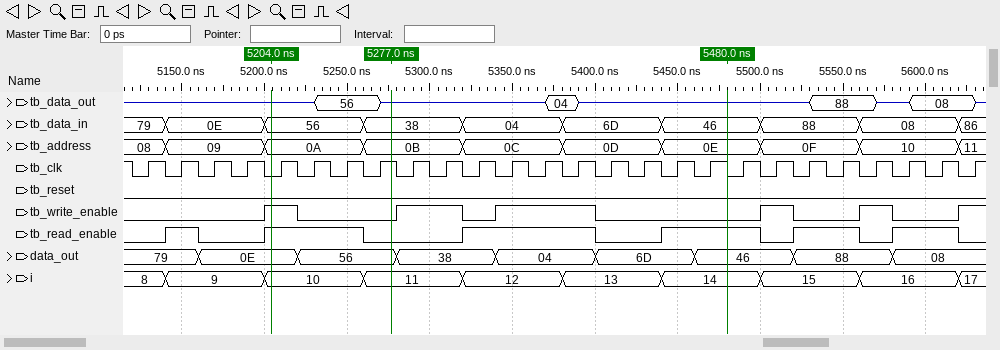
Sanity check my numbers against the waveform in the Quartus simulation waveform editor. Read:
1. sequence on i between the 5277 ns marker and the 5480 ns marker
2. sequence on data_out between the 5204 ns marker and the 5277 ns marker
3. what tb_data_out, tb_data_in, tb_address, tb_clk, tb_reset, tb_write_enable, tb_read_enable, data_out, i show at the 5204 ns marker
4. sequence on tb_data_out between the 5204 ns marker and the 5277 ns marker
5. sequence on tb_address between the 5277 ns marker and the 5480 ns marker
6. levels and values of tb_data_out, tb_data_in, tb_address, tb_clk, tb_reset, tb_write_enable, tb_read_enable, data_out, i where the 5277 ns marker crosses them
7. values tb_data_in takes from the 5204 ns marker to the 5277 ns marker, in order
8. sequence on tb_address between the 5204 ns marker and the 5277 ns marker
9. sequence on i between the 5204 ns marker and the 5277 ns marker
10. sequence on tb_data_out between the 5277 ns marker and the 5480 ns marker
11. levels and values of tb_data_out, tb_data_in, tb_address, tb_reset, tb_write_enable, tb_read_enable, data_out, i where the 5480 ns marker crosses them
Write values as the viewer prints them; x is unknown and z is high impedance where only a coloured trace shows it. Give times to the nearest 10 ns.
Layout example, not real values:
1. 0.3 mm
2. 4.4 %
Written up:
1. 11, 12, 13, 14
2. 0E, 56
3. tb_data_out=z, tb_data_in=56, tb_address=0A, tb_clk=0, tb_reset=0, tb_write_enable=1, tb_read_enable=1, data_out=0E, i=10
4. z, 56, z
5. 0B, 0C, 0D, 0E
6. tb_data_out=z, tb_data_in=38, tb_address=0B, tb_clk=1, tb_reset=0, tb_write_enable=0, tb_read_enable=0, data_out=56, i=11
7. 56, 38
8. 0A, 0B
9. 10, 11
10. z, 04, z
11. tb_data_out=z, tb_data_in=46, tb_address=0E, tb_reset=0, tb_write_enable=0, tb_read_enable=1, data_out=46, i=14
